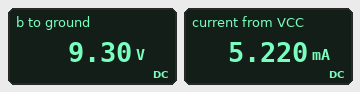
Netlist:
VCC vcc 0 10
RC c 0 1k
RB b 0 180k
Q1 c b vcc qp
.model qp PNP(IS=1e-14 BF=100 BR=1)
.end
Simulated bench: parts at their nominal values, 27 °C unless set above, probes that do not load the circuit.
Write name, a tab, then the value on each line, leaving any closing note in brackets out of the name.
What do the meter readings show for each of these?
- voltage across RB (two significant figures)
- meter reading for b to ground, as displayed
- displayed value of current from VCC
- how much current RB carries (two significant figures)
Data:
voltage across RB	9.3 V
meter reading for b to ground, as displayed	9.30 V
displayed value of current from VCC	5.220 mA
how much current RB carries	52 µA
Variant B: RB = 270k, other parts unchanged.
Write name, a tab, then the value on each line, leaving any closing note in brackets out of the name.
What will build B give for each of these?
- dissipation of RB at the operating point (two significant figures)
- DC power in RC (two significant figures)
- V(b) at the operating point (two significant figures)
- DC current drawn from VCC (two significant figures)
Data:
dissipation of RB at the operating point	320 µW
DC power in RC	12 mW
V(b) at the operating point	9.3 V
DC current drawn from VCC	3.5 mA
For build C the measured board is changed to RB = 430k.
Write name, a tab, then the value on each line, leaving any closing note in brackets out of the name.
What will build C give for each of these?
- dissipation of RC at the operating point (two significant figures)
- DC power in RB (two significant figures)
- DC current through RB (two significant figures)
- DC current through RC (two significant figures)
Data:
dissipation of RC at the operating point	4.7 mW
DC power in RB	200 µW
DC current through RB	22 µA
DC current through RC	2.2 mA
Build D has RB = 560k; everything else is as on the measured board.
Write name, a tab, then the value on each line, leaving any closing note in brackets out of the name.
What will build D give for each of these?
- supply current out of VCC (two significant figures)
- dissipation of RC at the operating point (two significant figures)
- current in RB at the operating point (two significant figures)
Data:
supply current out of VCC	1.7 mA
dissipation of RC at the operating point	2.8 mW
current in RB at the operating point	17 µA
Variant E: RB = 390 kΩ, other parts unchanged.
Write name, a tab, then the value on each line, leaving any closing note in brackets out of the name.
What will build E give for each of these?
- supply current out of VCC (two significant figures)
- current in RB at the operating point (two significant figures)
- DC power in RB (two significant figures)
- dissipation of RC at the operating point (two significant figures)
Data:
supply current out of VCC	2.4 mA
current in RB at the operating point	24 µA
DC power in RB	220 µW
dissipation of RC at the operating point	5.7 mW
